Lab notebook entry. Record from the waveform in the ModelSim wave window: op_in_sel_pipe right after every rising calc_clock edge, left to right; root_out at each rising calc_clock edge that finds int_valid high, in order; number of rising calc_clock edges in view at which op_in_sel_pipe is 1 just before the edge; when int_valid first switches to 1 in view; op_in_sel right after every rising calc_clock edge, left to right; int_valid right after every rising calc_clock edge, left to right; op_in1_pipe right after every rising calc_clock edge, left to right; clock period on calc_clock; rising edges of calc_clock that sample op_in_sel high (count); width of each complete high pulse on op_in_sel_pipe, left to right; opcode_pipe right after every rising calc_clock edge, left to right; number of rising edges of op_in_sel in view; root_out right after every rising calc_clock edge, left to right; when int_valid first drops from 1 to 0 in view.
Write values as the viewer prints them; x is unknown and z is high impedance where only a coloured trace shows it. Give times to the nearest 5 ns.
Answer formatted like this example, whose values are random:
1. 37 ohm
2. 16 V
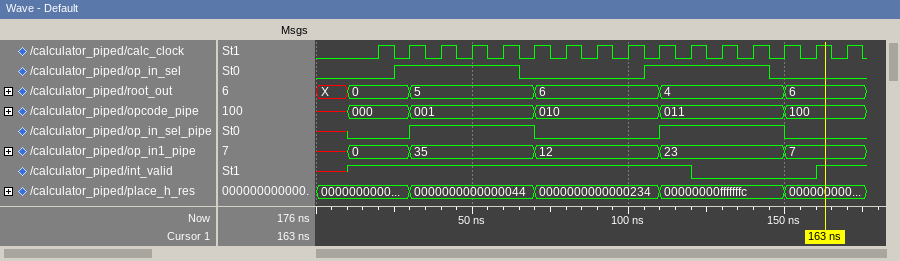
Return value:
1. 0 1 1 1 1 0 0 0 0 1 1 1 1 0 0 0
2. 0, 0, 5, 5, 5, 5, 6, 6, 6, 6, 4, 6
3. 8
4. 10 ns
5. 0 1 1 1 1 0 0 0 0 1 1 1 1 0 0 0
6. 1 1 1 1 1 1 1 1 1 1 0 0 0 0 1 1
7. 0, 35, 35, 35, 35, 12, 12, 12, 12, 23, 23, 23, 23, 7, 7, 7
8. 10 ns
9. 8
10. 40 ns, 40 ns
11. 000, 001, 001, 001, 001, 010, 010, 010, 010, 011, 011, 011, 011, 100, 100, 100
12. 2
13. 0, 5, 5, 5, 5, 6, 6, 6, 6, 4, 4, 4, 4, 6, 6, 6
14. 120 ns
